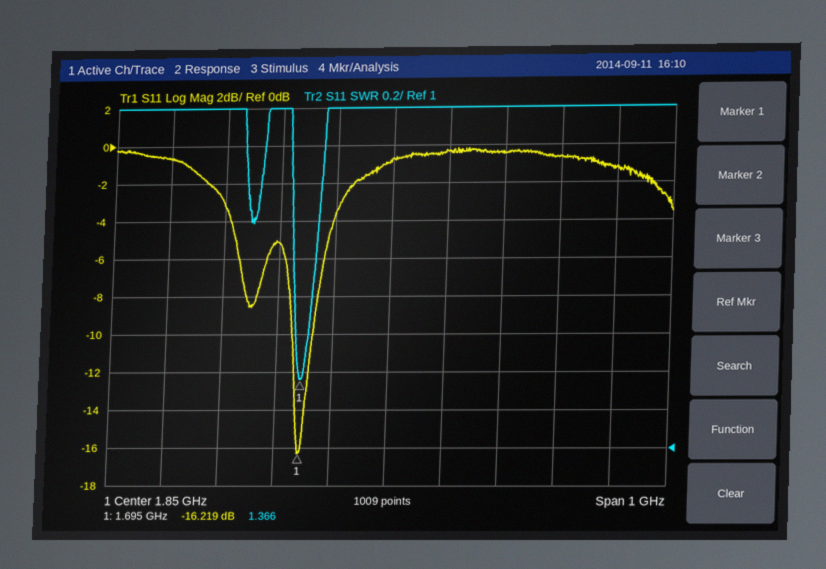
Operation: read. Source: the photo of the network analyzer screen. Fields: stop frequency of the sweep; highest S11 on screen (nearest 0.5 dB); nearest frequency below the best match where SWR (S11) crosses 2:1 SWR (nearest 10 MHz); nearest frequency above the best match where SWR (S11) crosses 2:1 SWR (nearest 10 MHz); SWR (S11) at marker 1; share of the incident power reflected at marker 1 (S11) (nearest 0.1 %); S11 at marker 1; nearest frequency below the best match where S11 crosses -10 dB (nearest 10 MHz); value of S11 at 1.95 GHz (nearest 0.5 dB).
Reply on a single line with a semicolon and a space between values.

2.35 GHz; 0.0 dB; 1.68 GHz; 1.72 GHz; 1.366; 2.4 %; -16.219 dB; 1.68 GHz; -0.5 dB
